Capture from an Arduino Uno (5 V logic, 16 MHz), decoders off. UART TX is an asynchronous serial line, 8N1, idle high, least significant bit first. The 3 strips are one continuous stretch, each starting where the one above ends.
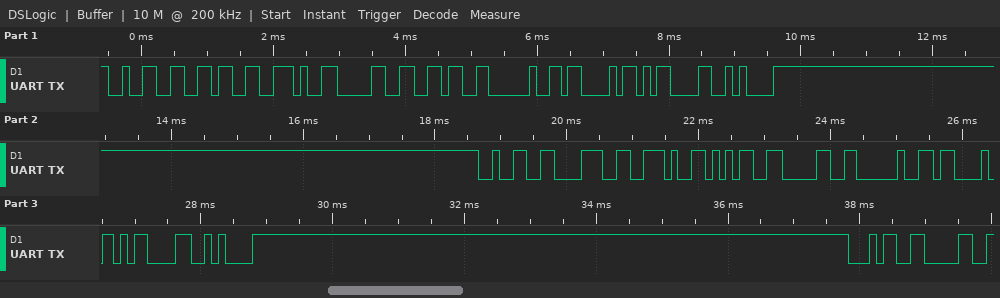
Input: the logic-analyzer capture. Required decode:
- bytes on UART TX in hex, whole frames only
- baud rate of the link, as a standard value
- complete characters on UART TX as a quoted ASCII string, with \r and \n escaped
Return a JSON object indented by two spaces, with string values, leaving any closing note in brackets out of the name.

{
  "bytes on UART TX in hex, whole frames only": "32 36 2E 30 36 20 43 0D 0A 32 38 2E 35 30 20 43 0D 0A 34 30",
  "baud rate of the link, as a standard value": "9600 baud",
  "complete characters on UART TX as a quoted ASCII string, with \\r and \\n escaped": "\"26.06 C\\r\\n28.50 C\\r\\n40\""
}
